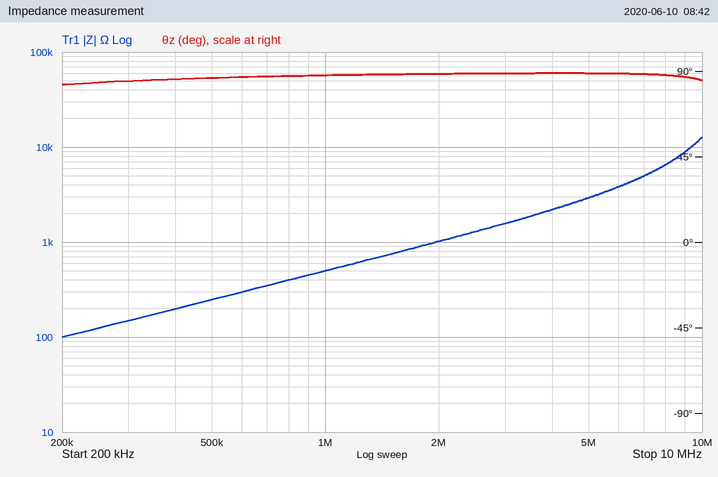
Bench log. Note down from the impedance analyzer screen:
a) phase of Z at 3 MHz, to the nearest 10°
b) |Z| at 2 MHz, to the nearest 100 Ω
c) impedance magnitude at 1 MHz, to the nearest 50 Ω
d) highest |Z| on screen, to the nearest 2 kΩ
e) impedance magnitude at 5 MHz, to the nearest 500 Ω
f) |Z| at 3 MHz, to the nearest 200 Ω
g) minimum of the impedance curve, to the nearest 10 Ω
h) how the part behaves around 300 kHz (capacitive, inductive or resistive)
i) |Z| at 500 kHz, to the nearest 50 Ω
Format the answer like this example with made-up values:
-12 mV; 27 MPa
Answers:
90°; 1.0 kΩ; 500 Ω; 12 kΩ; 3.0 kΩ; 1.6 kΩ; 100 Ω; inductive; 250 Ω
